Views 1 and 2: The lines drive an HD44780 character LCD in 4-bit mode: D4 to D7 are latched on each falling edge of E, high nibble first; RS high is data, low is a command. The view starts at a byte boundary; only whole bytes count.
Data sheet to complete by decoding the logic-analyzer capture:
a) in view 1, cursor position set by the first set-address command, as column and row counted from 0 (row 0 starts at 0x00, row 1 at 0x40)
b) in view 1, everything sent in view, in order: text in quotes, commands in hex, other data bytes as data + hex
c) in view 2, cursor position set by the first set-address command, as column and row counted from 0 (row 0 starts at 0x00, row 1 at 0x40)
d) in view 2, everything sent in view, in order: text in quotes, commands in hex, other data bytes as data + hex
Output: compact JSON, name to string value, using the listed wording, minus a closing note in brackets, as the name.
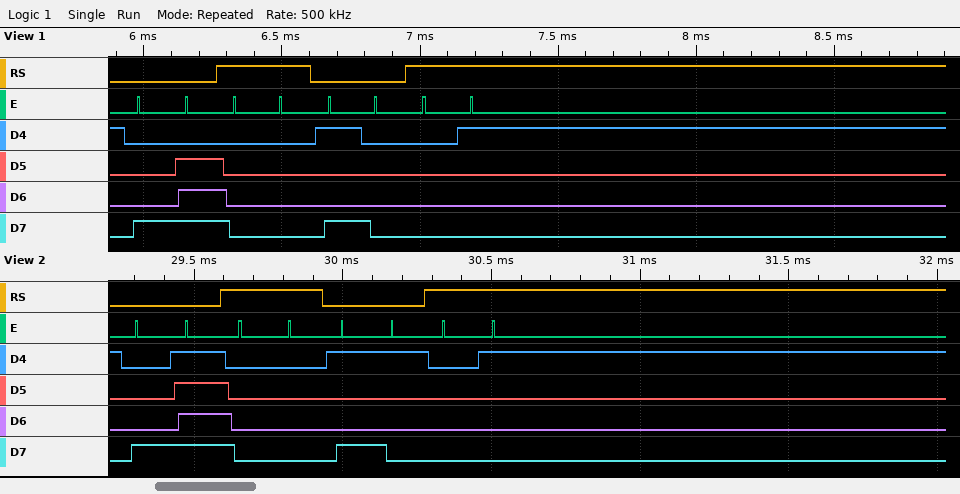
{"in view 1, cursor position set by the first set-address command, as column and row counted from 0": "column 14, row 0", "in view 1, everything sent in view, in order: text in quotes, commands in hex, other data bytes as data + hex": "0x8E data 00 0x90 data 01", "in view 2, cursor position set by the first set-address command, as column and row counted from 0": "column 15, row 0", "in view 2, everything sent in view, in order: text in quotes, commands in hex, other data bytes as data + hex": "0x8F data 00 0x91 data 01"}
